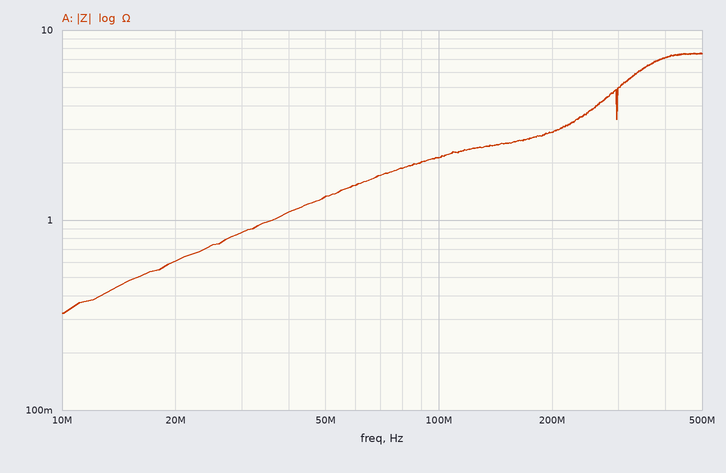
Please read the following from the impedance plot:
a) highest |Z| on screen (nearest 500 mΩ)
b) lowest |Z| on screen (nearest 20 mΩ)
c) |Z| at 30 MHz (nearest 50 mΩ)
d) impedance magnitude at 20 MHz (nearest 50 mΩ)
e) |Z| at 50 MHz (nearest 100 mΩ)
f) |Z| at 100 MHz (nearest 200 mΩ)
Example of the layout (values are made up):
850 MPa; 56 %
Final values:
7.5 Ω; 320 mΩ; 850 mΩ; 600 mΩ; 1.3 Ω; 2.2 Ω
